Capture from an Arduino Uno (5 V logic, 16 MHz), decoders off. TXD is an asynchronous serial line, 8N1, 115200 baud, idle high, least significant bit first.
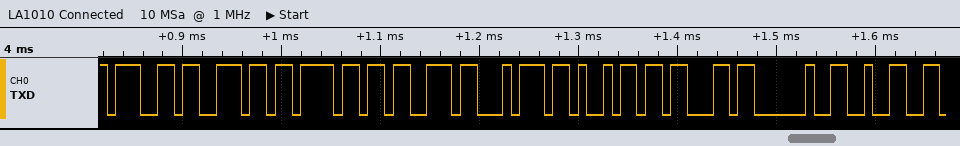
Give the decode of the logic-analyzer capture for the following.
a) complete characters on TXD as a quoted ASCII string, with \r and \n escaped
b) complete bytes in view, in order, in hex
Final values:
"gnostic 2"
0x67 0x6E 0x6F 0x73 0x74 0x69 0x63 0x20 0x32
